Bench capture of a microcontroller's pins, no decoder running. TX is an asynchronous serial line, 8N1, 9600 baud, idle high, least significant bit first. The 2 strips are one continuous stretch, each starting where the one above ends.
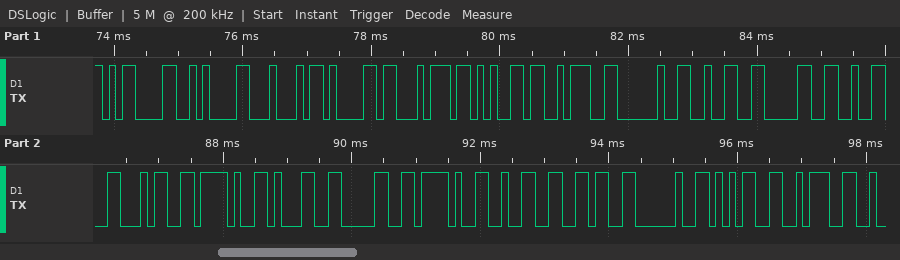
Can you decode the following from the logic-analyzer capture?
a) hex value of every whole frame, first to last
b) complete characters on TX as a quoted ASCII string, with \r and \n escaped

0x0D 0x0A 0x44 0x61 0x74 0x65 0x3A 0x20 0x32 0x30 0x32 0x34 0x2F 0x31 0x30 0x2F 0x32 0x36 0x20 0x35 0x3A
"\r\nDate: 2024/10/26 5:"
